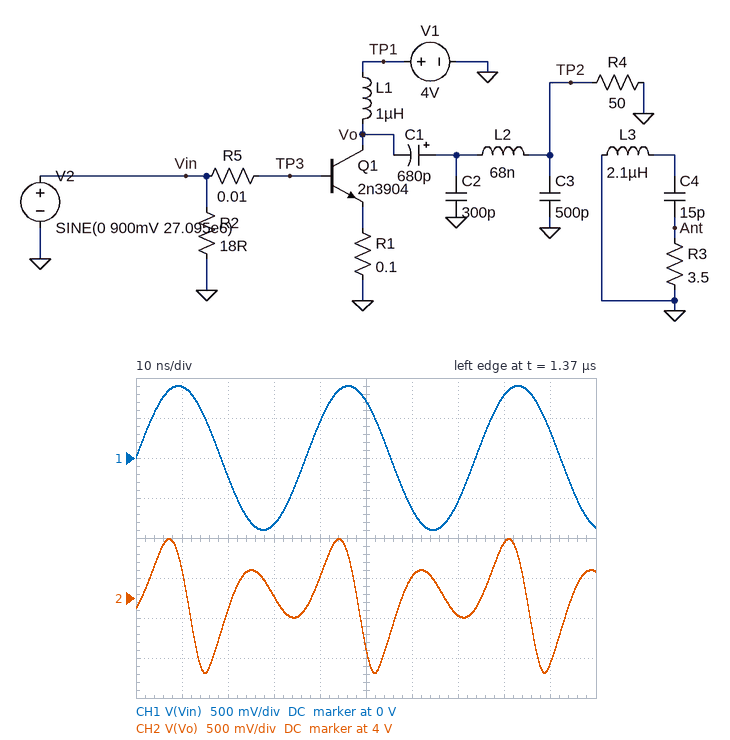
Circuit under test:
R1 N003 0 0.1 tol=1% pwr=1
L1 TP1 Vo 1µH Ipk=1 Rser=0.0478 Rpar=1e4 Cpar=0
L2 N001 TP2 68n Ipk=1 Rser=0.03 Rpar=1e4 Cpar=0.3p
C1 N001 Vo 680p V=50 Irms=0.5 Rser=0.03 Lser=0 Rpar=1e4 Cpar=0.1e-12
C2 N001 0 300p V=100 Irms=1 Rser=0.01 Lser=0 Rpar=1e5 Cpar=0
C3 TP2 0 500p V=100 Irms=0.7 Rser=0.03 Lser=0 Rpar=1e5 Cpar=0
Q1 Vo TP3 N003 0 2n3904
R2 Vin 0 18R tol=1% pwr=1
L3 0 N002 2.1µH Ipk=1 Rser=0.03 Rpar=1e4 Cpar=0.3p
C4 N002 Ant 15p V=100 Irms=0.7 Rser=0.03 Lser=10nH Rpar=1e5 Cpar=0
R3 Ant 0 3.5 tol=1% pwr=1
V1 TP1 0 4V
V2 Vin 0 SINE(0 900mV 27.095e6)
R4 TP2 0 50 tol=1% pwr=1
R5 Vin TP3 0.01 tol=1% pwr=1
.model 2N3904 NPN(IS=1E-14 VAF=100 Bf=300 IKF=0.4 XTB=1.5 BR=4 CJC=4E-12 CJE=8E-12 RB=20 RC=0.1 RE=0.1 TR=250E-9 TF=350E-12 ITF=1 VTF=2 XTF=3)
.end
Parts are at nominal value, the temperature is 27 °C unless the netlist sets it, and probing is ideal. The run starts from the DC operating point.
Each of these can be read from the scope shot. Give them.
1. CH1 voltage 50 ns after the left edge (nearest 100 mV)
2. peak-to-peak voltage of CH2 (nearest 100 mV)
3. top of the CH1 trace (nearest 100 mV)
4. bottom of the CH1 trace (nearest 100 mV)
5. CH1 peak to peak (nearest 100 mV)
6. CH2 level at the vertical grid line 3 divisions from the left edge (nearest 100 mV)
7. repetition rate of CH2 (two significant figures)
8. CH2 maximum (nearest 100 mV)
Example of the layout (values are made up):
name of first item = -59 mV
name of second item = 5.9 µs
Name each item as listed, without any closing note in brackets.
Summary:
CH1 voltage 50 ns after the left edge = 700 mV
peak-to-peak voltage of CH2 = 1.7 V
top of the CH1 trace = 900 mV
bottom of the CH1 trace = -900 mV
CH1 peak to peak = 1.8 V
CH2 level at the vertical grid line 3 divisions from the left edge = 4.0 V
repetition rate of CH2 = 27 MHz
CH2 maximum = 4.7 V
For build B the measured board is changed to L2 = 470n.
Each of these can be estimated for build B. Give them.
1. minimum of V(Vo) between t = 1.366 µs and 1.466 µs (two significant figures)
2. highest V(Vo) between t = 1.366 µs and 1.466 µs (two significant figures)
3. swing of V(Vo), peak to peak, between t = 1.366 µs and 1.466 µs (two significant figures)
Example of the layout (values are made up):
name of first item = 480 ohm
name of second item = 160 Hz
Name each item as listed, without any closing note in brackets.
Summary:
minimum of V(Vo) between t = 1.366 µs and 1.466 µs = 2.9 V
highest V(Vo) between t = 1.366 µs and 1.466 µs = 5.1 V
swing of V(Vo), peak to peak, between t = 1.366 µs and 1.466 µs = 2.2 V
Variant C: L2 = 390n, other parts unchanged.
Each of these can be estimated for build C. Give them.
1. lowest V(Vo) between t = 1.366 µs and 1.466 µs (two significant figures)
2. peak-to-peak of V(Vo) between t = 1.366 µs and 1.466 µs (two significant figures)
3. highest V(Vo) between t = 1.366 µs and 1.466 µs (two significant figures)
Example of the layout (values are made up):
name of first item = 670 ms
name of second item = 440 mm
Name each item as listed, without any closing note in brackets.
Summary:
lowest V(Vo) between t = 1.366 µs and 1.466 µs = 2.8 V
peak-to-peak of V(Vo) between t = 1.366 µs and 1.466 µs = 2.4 V
highest V(Vo) between t = 1.366 µs and 1.466 µs = 5.2 V
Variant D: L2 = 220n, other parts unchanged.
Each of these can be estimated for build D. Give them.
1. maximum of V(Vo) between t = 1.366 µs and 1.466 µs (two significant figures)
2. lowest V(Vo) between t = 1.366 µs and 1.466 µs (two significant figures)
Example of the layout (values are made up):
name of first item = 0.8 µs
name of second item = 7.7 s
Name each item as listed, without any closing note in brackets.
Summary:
maximum of V(Vo) between t = 1.366 µs and 1.466 µs = 6.5 V
lowest V(Vo) between t = 1.366 µs and 1.466 µs = 1.1 V
